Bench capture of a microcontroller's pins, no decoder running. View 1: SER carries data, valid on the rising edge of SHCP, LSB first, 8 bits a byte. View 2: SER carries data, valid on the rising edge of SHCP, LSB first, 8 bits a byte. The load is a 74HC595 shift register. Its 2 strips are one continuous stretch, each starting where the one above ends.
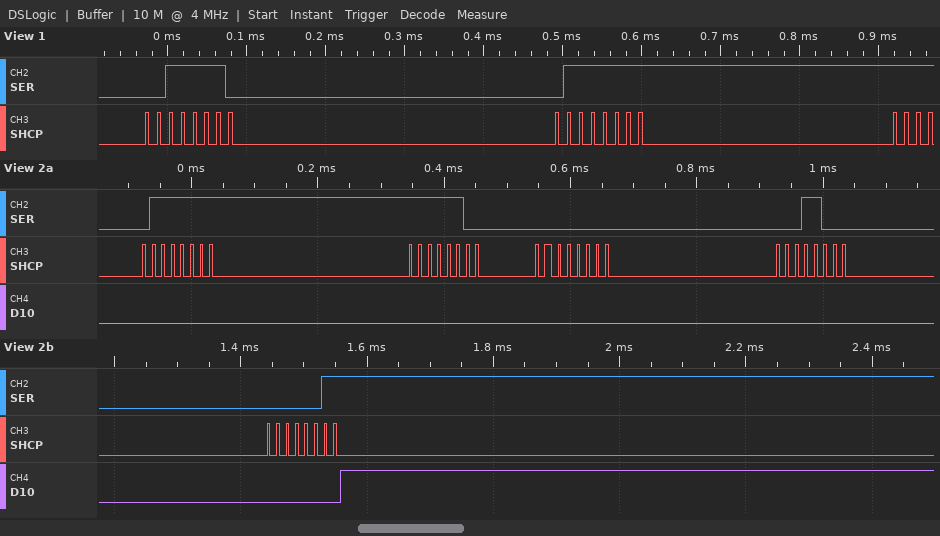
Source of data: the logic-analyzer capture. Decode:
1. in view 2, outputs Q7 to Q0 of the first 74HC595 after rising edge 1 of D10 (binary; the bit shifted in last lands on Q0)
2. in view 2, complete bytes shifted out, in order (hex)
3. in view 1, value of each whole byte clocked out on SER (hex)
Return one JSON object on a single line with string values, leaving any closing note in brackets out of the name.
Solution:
{"in view 2, outputs Q7 to Q0 of the first 74HC595 after rising edge 1 of D10": "00000011", "in view 2, complete bytes shifted out, in order": "0xFE 0x3F 0x00 0x18 0xC0", "in view 1, value of each whole byte clocked out on SER": "7C FE"}
